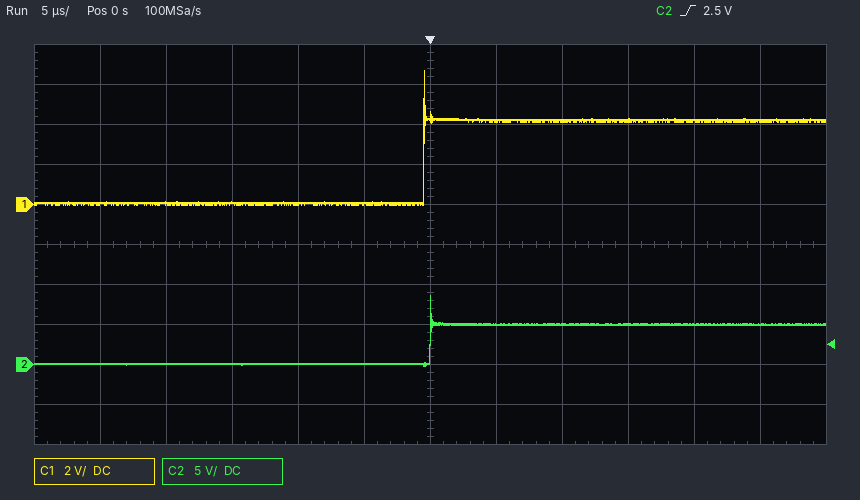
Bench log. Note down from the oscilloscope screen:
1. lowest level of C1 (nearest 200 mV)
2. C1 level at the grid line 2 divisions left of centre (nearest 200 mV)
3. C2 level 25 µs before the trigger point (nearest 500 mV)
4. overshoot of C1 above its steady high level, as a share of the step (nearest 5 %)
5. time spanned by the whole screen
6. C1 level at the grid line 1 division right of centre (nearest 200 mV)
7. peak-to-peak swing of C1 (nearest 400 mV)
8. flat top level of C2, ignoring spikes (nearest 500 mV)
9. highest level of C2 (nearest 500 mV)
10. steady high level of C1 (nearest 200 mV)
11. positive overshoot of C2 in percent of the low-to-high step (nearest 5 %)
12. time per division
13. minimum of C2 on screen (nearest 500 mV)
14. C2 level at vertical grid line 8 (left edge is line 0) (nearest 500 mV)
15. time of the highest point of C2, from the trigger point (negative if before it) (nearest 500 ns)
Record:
0.0 V
0.0 V
0.0 V
60 %
60 µs
4.2 V
6.8 V
5.0 V
8.5 V
4.2 V
70 %
5 µs
0.0 V
5.0 V
0.0 µs
